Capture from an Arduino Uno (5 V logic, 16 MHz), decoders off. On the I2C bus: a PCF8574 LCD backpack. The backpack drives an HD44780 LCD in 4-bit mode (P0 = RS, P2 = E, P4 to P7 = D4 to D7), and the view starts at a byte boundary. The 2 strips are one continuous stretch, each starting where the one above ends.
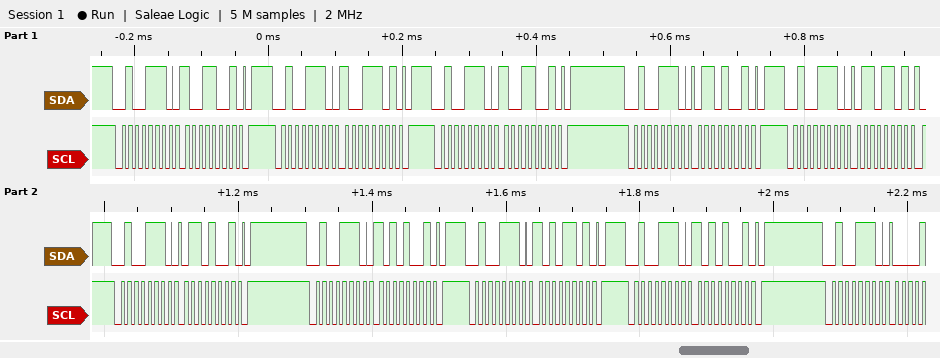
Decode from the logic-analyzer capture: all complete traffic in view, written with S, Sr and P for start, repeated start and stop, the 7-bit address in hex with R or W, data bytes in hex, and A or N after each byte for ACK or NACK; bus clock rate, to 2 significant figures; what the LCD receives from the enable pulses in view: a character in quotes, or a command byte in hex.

S 27W A 99 A P S 27W A 9D A P S 27W A 99 A P S 27W A 69 A P S 27W A 6D A P S 27W A 69 A P S 27W A A9 A P S 27W A AD A P S 27W A A9 A P S 27W A
100 kHz
data 0x96
